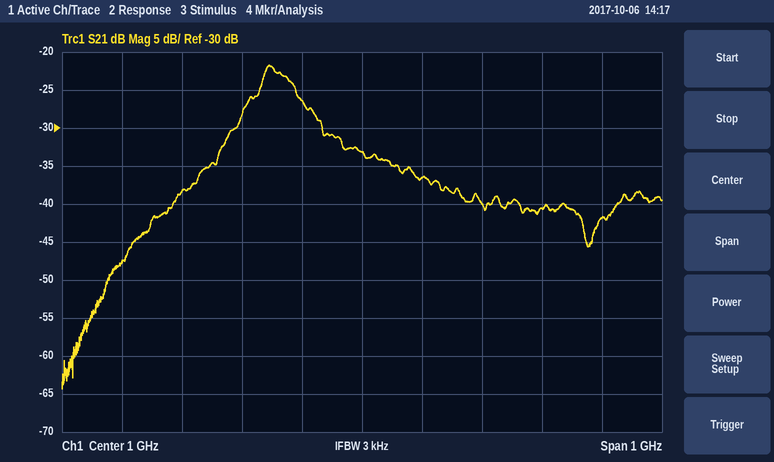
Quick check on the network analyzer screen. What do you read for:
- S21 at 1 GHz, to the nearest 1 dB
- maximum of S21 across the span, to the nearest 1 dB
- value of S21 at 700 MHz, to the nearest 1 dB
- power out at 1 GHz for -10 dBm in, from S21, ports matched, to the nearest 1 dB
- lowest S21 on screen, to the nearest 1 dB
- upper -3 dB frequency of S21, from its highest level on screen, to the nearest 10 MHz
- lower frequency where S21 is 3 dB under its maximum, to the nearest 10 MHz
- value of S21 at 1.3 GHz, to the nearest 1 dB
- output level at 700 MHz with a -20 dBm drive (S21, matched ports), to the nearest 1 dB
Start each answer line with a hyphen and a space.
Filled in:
- -33 dB
- -22 dB
- -38 dB
- -43 dBm
- -64 dB
- 890 MHz
- 830 MHz
- -41 dB
- -58 dBm
